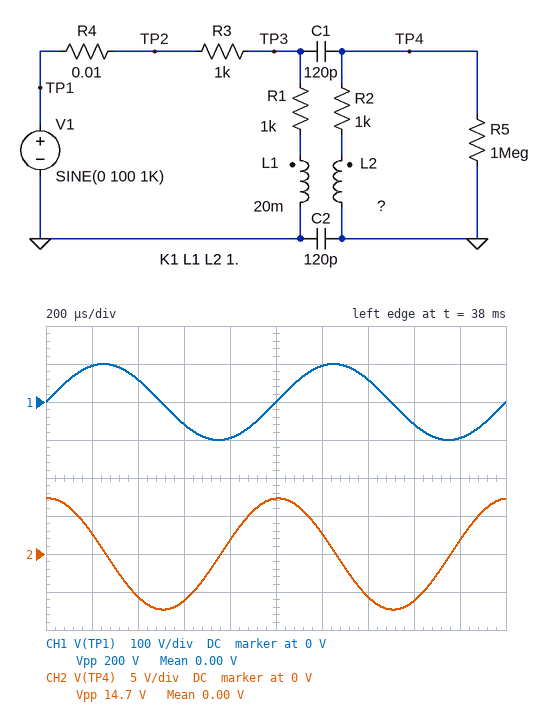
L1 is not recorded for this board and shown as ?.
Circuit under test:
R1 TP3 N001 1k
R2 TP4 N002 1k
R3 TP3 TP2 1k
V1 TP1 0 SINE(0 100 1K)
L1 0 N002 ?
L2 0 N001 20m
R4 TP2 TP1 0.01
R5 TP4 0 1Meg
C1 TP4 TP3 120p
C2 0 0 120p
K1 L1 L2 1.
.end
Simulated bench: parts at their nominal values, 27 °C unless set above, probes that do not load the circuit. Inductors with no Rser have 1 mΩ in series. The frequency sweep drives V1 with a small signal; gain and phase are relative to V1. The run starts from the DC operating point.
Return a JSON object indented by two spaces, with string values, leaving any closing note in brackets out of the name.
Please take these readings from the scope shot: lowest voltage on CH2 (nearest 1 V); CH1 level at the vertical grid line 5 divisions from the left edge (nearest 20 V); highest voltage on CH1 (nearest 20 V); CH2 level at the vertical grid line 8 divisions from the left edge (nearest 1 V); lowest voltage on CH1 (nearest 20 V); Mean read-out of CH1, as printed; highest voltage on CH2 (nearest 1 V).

{
  "lowest voltage on CH2": "-7 V",
  "CH1 level at the vertical grid line 5 divisions from the left edge": "0 V",
  "highest voltage on CH1": "100 V",
  "CH2 level at the vertical grid line 8 divisions from the left edge": "-6 V",
  "lowest voltage on CH1": "-100 V",
  "Mean read-out of CH1, as printed": "0.00 V",
  "highest voltage on CH2": "7 V"
}
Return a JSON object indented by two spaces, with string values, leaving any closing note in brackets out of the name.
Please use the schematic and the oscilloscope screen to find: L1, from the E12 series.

{
  "L1, from the E12 series": "27 mH"
}
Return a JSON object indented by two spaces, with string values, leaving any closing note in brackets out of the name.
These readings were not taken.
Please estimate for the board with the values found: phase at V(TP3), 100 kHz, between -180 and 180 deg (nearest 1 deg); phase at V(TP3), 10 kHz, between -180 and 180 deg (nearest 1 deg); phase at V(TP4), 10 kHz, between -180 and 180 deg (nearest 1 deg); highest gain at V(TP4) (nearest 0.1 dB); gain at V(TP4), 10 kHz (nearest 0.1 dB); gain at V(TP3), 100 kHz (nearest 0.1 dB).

{
  "phase at V(TP3), 100 kHz, between -180 and 180 deg": "4 deg",
  "phase at V(TP3), 10 kHz, between -180 and 180 deg": "19 deg",
  "phase at V(TP4), 10 kHz, between -180 and 180 deg": "58 deg",
  "highest gain at V(TP4)": "1.3 dB",
  "gain at V(TP4), 10 kHz": "-4.1 dB",
  "gain at V(TP3), 100 kHz": "-0.1 dB"
}
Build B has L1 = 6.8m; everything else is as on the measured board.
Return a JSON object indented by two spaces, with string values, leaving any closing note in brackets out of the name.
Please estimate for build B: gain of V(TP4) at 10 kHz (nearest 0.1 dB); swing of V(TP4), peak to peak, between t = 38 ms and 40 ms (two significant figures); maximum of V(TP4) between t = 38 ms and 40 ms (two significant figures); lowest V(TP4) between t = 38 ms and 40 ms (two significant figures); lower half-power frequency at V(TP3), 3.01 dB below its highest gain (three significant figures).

{
  "gain of V(TP4) at 10 kHz": "-10.1 dB",
  "swing of V(TP4), peak to peak, between t = 38 ms and 40 ms": "7.4 V",
  "maximum of V(TP4) between t = 38 ms and 40 ms": "3.7 V",
  "lowest V(TP4) between t = 38 ms and 40 ms": "-3.7 V",
  "lower half-power frequency at V(TP3), 3.01 dB below its highest gain": "11.0 kHz"
}
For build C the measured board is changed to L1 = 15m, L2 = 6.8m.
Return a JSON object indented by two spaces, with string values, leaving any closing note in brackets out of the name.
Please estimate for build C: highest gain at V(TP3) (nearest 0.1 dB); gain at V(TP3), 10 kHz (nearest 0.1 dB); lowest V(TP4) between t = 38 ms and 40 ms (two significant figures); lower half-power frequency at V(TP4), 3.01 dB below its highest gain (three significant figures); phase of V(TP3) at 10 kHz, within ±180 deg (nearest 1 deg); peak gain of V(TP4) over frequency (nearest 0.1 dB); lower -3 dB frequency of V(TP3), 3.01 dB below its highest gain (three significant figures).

{
  "highest gain at V(TP3)": "-0.1 dB",
  "gain at V(TP3), 10 kHz": "-5.5 dB",
  "lowest V(TP4) between t = 38 ms and 40 ms": "-3.2 V",
  "lower half-power frequency at V(TP4), 3.01 dB below its highest gain": "41.9 kHz",
  "phase of V(TP3) at 10 kHz, within ±180 deg": "11 deg",
  "peak gain of V(TP4) over frequency": "3.3 dB",
  "lower -3 dB frequency of V(TP3), 3.01 dB below its highest gain": "32.4 kHz"
}
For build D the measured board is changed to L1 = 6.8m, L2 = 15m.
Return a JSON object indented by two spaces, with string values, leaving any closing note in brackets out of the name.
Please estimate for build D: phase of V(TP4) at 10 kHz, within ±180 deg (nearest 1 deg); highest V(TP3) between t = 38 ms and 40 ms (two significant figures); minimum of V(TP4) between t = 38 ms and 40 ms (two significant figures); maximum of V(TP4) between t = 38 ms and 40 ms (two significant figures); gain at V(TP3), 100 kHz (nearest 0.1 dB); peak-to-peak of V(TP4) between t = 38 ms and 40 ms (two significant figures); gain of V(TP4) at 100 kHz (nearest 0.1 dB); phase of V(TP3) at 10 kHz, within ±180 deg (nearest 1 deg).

{
  "phase of V(TP4) at 10 kHz, within ±180 deg": "65 deg",
  "highest V(TP3) between t = 38 ms and 40 ms": "50 V",
  "minimum of V(TP4) between t = 38 ms and 40 ms": "-3.2 V",
  "maximum of V(TP4) between t = 38 ms and 40 ms": "3.2 V",
  "gain at V(TP3), 100 kHz": "-0.2 dB",
  "peak-to-peak of V(TP4) between t = 38 ms and 40 ms": "6.4 V",
  "gain of V(TP4) at 100 kHz": "-3.5 dB",
  "phase of V(TP3) at 10 kHz, within ±180 deg": "18 deg"
}
